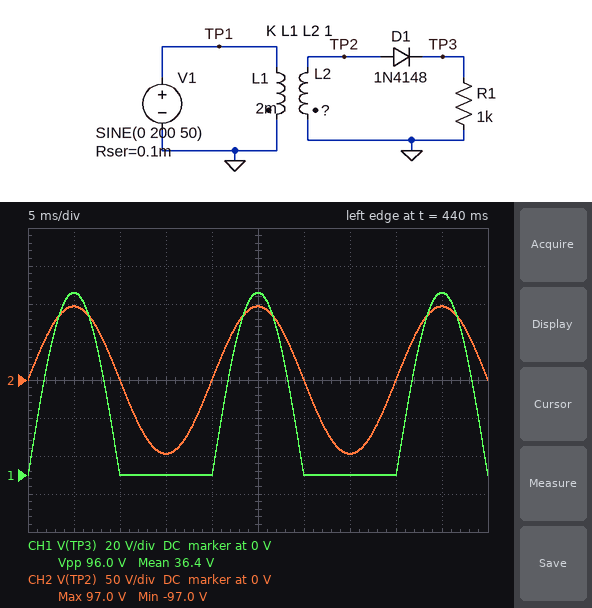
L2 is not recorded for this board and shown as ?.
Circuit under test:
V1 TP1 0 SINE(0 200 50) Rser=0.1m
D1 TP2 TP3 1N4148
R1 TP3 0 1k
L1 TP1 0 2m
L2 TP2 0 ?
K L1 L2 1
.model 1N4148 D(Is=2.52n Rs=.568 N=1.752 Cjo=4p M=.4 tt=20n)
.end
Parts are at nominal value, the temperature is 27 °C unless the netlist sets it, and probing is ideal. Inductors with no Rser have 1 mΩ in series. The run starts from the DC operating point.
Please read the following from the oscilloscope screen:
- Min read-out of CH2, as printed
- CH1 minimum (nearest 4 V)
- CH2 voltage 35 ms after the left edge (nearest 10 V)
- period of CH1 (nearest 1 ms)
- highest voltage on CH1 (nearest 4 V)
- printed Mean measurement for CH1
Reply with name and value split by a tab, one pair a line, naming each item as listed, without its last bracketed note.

Min read-out of CH2, as printed	-97.0 V
CH1 minimum	0 V
CH2 voltage 35 ms after the left edge	-100 V
period of CH1	20 ms
highest voltage on CH1	96 V
printed Mean measurement for CH1	36.4 V
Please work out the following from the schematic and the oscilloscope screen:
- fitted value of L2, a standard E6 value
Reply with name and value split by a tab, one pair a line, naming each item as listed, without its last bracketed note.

fitted value of L2, a standard E6 value	470 µH
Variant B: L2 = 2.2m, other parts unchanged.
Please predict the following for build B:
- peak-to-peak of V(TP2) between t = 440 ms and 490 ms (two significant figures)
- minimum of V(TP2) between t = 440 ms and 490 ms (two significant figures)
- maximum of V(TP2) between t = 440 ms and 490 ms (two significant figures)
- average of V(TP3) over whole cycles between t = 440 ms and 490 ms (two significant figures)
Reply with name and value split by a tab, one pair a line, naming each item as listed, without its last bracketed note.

peak-to-peak of V(TP2) between t = 440 ms and 490 ms	420 V
minimum of V(TP2) between t = 440 ms and 490 ms	-210 V
maximum of V(TP2) between t = 440 ms and 490 ms	210 V
average of V(TP3) over whole cycles between t = 440 ms and 490 ms	66 V
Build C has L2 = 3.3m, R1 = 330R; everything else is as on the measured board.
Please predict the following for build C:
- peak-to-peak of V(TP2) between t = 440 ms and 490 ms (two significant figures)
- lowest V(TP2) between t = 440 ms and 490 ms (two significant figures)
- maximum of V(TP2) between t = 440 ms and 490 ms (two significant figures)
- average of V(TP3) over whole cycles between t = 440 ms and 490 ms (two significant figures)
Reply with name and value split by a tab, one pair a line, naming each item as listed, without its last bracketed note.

peak-to-peak of V(TP2) between t = 440 ms and 490 ms	510 V
lowest V(TP2) between t = 440 ms and 490 ms	-260 V
maximum of V(TP2) between t = 440 ms and 490 ms	260 V
average of V(TP3) over whole cycles between t = 440 ms and 490 ms	81 V
